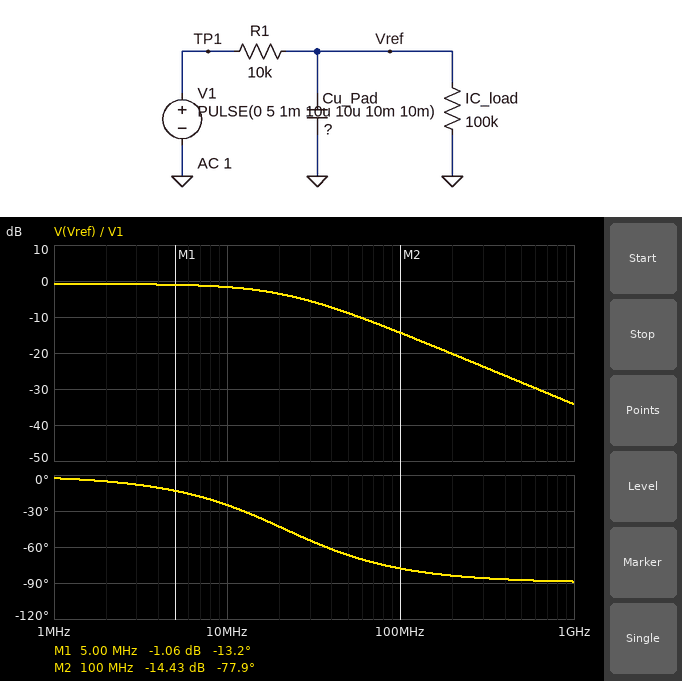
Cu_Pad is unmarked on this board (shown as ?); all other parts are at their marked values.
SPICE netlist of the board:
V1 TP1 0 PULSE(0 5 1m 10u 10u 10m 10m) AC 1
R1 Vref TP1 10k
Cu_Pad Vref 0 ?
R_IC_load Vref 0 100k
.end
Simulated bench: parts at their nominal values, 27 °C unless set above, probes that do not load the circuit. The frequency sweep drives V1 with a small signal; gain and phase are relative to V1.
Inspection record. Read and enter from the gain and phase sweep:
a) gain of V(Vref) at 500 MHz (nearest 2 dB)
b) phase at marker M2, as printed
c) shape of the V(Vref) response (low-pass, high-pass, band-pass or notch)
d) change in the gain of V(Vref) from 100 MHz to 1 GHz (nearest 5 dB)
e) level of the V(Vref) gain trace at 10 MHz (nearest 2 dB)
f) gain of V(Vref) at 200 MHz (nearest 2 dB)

-28 dB
-77.9 deg
low-pass
-20 dB
-2 dB
-20 dB
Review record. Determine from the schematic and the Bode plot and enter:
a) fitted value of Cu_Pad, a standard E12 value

820 fF
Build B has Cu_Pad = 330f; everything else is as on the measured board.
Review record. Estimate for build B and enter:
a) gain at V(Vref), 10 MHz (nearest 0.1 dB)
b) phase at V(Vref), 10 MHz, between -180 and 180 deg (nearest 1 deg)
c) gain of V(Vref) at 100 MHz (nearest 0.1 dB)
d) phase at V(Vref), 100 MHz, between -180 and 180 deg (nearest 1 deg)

-1.0 dB
-11 deg
-7.4 dB
-62 deg
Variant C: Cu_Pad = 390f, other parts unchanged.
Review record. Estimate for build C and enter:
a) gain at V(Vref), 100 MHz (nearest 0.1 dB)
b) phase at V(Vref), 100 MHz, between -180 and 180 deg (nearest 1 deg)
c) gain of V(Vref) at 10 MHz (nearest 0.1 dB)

-8.6 dB
-66 deg
-1.0 dB
